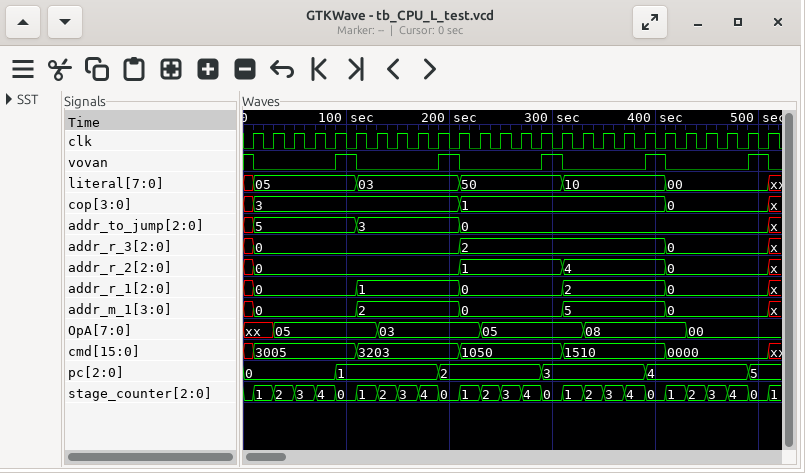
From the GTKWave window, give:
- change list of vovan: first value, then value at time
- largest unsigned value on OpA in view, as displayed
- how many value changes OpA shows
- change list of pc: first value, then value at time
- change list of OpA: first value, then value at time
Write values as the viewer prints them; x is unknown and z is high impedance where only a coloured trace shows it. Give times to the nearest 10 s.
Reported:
1, 0 at 10 s, 1 at 90 s, 0 at 110 s, 1 at 190 s, 0 at 210 s, 1 at 290 s, 0 at 310 s, 1 at 390 s, 0 at 410 s, 1 at 490 s, 0 at 510 s
08
5
0, 1 at 90 s, 2 at 190 s, 3 at 290 s, 4 at 390 s, 5 at 490 s
xx, 05 at 30 s, 03 at 130 s, 05 at 230 s, 08 at 330 s, 00 at 430 s
